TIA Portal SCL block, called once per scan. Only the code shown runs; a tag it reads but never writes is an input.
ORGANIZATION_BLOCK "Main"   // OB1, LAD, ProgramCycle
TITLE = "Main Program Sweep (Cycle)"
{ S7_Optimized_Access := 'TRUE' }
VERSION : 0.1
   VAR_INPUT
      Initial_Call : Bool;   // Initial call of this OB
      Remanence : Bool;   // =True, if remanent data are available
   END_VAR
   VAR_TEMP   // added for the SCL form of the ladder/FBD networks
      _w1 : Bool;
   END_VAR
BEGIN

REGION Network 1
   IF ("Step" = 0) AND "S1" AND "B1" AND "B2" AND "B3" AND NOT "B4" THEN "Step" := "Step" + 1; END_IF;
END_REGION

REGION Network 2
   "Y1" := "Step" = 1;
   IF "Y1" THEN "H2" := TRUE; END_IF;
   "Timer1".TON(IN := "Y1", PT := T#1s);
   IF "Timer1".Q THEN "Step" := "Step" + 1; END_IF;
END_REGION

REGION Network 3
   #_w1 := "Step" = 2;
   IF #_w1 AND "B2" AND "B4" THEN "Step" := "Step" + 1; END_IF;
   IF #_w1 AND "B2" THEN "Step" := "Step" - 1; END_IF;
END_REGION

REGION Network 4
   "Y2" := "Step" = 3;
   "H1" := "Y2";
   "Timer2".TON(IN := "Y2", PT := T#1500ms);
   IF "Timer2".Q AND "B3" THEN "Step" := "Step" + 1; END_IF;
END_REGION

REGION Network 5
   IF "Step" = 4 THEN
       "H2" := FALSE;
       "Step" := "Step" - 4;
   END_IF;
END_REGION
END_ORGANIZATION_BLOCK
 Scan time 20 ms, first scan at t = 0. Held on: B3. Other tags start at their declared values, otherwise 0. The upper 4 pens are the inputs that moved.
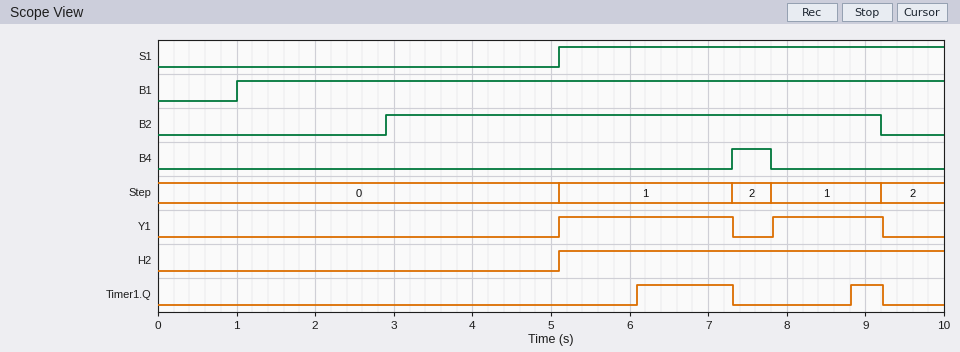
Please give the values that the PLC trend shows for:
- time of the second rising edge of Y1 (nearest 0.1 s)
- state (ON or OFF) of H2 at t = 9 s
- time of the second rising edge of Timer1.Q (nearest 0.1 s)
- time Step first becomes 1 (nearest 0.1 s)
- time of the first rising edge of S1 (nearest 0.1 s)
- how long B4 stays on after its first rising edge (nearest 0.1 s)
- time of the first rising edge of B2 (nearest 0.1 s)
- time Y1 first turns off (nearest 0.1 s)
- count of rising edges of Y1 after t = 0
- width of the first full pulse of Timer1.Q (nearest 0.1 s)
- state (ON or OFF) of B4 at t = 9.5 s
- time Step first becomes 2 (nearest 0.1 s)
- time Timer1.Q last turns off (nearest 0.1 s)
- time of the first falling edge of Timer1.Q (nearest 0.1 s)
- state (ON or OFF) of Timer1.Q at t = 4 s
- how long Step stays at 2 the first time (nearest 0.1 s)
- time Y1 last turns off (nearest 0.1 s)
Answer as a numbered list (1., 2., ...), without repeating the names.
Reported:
1. 7.8 s
2. ON
3. 8.8 s
4. 5.1 s
5. 5.1 s
6. 0.5 s
7. 2.9 s
8. 7.3 s
9. 2
10. 1.2 s
11. OFF
12. 7.3 s
13. 9.2 s
14. 7.3 s
15. OFF
16. 0.5 s
17. 9.2 s
